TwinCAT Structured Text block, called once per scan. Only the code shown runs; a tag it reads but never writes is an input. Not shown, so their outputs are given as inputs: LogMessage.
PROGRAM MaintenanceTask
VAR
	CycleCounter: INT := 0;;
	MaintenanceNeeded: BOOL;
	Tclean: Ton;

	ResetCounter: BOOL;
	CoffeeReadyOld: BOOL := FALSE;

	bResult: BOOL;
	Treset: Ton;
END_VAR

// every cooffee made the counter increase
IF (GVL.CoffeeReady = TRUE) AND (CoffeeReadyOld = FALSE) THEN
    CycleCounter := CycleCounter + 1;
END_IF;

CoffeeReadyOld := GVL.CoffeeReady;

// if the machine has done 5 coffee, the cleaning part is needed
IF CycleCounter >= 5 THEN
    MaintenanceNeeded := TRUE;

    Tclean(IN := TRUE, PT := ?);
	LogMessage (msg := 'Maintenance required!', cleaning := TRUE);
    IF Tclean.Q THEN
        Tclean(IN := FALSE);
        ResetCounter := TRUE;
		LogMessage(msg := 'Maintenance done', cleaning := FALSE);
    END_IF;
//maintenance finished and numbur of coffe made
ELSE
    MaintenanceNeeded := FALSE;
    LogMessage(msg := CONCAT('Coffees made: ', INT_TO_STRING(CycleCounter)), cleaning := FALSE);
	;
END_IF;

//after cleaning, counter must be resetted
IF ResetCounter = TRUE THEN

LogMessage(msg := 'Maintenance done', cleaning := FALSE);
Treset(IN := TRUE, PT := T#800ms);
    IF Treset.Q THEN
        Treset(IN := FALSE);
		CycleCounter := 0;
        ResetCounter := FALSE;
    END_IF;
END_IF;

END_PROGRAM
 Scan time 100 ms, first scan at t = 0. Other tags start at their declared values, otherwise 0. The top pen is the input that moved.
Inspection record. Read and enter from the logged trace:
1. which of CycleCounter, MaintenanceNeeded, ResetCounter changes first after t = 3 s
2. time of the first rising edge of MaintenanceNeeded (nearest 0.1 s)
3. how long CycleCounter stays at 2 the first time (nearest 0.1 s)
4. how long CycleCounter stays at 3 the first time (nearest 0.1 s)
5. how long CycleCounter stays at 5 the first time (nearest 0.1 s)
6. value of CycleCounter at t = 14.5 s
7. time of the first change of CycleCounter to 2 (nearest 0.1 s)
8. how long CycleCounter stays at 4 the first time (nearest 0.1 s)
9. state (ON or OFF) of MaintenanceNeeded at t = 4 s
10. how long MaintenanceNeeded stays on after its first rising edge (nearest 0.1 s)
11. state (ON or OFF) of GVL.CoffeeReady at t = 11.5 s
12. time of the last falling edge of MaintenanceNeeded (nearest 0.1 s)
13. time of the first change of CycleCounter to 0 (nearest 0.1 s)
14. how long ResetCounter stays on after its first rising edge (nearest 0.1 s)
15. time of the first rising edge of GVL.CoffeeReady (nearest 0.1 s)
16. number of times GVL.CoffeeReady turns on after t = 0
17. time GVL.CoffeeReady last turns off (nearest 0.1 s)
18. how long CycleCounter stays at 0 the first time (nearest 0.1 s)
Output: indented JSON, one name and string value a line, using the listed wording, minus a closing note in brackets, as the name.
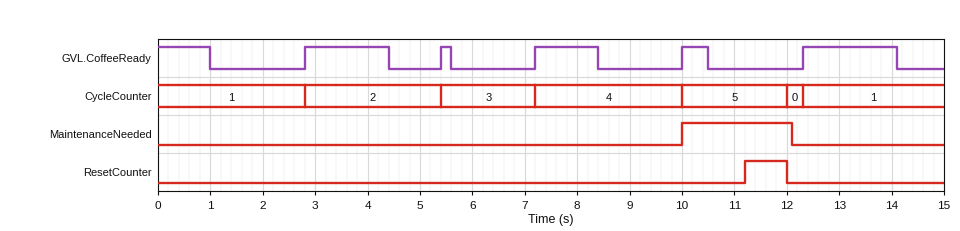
{
  "which of CycleCounter, MaintenanceNeeded, ResetCounter changes first after t = 3 s": "CycleCounter",
  "time of the first rising edge of MaintenanceNeeded": "10.0 s",
  "how long CycleCounter stays at 2 the first time": "2.6 s",
  "how long CycleCounter stays at 3 the first time": "1.8 s",
  "how long CycleCounter stays at 5 the first time": "2.0 s",
  "value of CycleCounter at t = 14.5 s": "1",
  "time of the first change of CycleCounter to 2": "2.8 s",
  "how long CycleCounter stays at 4 the first time": "2.8 s",
  "state (ON or OFF) of MaintenanceNeeded at t = 4 s": "OFF",
  "how long MaintenanceNeeded stays on after its first rising edge": "2.1 s",
  "state (ON or OFF) of GVL.CoffeeReady at t = 11.5 s": "OFF",
  "time of the last falling edge of MaintenanceNeeded": "12.1 s",
  "time of the first change of CycleCounter to 0": "12.0 s",
  "how long ResetCounter stays on after its first rising edge": "0.8 s",
  "time of the first rising edge of GVL.CoffeeReady": "2.8 s",
  "number of times GVL.CoffeeReady turns on after t = 0": "5",
  "time GVL.CoffeeReady last turns off": "14.1 s",
  "how long CycleCounter stays at 0 the first time": "0.3 s"
}
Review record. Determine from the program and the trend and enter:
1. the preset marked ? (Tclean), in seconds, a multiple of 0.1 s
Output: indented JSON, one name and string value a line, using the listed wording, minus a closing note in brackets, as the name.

{
  "the preset marked ? (Tclean), in seconds, a multiple of 0.1 s": "1.2 s"
}
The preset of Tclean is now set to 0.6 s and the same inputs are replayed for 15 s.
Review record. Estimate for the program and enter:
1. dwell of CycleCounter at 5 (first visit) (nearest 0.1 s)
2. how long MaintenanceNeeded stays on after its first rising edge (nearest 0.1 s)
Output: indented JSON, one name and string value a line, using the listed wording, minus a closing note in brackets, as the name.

{
  "dwell of CycleCounter at 5 (first visit)": "1.4 s",
  "how long MaintenanceNeeded stays on after its first rising edge": "1.5 s"
}
